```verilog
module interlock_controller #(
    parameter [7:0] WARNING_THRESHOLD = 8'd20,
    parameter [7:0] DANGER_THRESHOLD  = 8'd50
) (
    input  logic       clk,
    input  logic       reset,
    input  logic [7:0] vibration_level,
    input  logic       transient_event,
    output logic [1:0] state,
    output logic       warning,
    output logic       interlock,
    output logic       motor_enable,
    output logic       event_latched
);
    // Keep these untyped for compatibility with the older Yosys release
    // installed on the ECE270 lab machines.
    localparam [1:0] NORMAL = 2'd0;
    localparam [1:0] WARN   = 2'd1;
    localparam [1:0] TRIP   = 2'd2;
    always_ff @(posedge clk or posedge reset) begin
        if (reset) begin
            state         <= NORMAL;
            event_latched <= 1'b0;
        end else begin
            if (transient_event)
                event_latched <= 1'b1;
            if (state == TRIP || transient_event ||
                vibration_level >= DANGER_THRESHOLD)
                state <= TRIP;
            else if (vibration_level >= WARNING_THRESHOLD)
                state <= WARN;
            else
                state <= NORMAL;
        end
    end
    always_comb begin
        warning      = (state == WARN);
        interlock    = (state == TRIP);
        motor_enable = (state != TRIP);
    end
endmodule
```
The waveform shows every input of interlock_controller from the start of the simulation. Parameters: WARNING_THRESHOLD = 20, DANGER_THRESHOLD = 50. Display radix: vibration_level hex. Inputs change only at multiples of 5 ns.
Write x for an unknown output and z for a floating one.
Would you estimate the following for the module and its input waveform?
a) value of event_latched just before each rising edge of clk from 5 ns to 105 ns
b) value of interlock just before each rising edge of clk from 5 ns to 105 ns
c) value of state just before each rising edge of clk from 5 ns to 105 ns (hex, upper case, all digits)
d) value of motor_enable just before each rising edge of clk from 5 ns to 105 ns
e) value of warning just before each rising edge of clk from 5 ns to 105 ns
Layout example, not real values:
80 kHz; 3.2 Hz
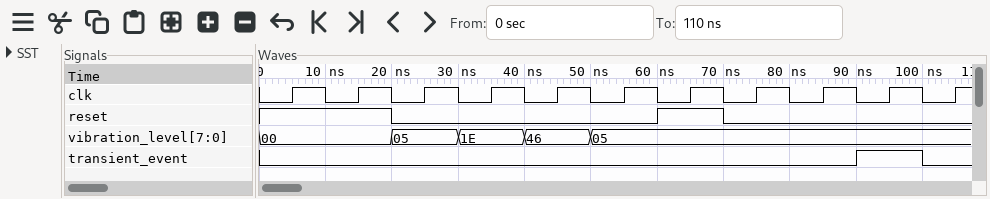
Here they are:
0 0 0 0 0 0 0 0 0 0 1; 0 0 0 0 0 1 0 0 0 0 1; 0, 0, 0, 0, 1, 2, 0, 0, 0, 0, 2; 1 1 1 1 1 0 1 1 1 1 0; 0 0 0 0 1 0 0 0 0 0 0
